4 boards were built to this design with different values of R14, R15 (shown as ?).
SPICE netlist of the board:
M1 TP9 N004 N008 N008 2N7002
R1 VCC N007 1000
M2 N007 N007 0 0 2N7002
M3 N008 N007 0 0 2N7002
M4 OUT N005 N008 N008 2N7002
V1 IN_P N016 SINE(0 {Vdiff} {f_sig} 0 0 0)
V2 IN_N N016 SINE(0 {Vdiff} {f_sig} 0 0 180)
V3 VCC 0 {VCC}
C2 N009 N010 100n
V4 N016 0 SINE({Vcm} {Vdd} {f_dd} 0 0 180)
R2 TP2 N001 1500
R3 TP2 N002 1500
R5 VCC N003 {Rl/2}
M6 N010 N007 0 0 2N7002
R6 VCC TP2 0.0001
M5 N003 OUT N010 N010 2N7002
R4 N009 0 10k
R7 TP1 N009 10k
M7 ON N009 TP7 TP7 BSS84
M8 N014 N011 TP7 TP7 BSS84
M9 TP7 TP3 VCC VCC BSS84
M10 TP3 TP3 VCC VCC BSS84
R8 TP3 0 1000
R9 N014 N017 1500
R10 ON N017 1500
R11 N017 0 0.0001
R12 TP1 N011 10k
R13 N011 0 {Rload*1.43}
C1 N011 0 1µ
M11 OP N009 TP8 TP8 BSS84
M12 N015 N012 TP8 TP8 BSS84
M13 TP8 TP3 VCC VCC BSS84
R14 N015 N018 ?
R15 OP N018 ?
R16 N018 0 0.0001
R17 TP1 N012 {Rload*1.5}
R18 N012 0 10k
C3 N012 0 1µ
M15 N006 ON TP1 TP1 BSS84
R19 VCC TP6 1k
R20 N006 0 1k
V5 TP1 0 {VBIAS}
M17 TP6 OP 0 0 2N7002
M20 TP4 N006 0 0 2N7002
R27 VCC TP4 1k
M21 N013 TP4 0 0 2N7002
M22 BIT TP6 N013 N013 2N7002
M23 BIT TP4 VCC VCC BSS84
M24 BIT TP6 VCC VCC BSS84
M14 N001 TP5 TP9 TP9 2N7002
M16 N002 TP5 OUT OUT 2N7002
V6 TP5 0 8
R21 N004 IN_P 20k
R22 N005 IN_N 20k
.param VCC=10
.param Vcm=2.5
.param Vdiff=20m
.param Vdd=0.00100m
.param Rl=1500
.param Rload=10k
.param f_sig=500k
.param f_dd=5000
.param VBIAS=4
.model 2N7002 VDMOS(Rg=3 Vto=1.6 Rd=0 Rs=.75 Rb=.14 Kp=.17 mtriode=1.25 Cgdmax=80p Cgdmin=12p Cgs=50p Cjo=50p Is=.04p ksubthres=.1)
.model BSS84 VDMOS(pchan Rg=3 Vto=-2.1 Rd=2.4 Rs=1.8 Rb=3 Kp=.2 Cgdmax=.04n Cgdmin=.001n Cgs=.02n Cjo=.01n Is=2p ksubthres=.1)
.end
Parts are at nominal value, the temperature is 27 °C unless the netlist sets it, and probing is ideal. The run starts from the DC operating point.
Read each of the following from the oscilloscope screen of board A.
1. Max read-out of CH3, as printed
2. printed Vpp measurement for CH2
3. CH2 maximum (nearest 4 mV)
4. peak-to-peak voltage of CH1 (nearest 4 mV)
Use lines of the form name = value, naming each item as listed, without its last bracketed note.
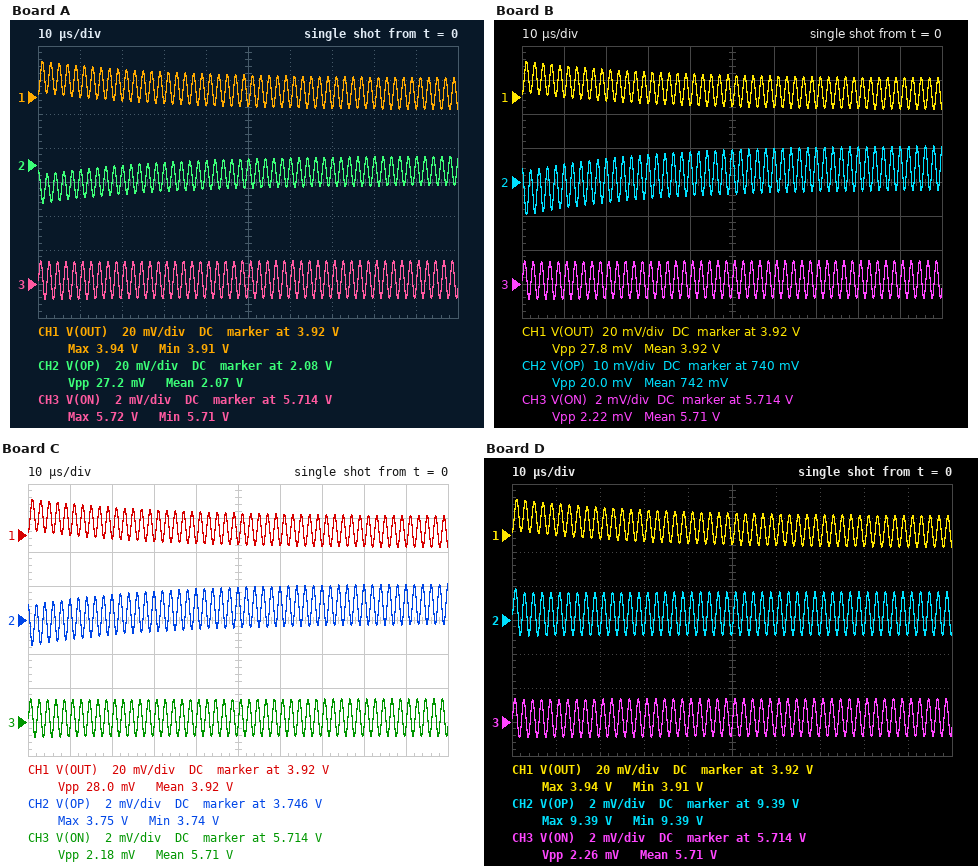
Max read-out of CH3, as printed = 5.72 V
printed Vpp measurement for CH2 = 27.2 mV
CH2 maximum = 2.084 V
peak-to-peak voltage of CH1 = 28 mV
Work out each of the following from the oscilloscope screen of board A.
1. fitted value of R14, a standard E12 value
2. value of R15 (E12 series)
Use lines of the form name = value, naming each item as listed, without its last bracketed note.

fitted value of R14, a standard E12 value = 820 Ω
value of R15 = 820 Ω
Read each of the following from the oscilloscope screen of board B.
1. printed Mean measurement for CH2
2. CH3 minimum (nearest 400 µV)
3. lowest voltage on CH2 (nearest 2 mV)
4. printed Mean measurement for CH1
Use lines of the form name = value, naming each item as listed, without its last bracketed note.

printed Mean measurement for CH2 = 742 mV
CH3 minimum = 5.7132 V
lowest voltage on CH2 = 730 mV
printed Mean measurement for CH1 = 3.92 V
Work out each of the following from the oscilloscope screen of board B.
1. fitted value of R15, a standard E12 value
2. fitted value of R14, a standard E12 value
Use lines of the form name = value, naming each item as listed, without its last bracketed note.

fitted value of R15, a standard E12 value = 470 Ω
fitted value of R14, a standard E12 value = 680 Ω
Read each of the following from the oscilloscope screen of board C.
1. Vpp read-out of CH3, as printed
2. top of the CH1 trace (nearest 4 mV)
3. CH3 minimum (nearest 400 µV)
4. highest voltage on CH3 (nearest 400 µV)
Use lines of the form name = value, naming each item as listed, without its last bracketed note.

Vpp read-out of CH3, as printed = 2.18 mV
top of the CH1 trace = 3.940 V
CH3 minimum = 5.7132 V
highest voltage on CH3 = 5.7152 V
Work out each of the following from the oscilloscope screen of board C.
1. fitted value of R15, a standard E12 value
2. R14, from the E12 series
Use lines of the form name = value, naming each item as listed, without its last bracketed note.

fitted value of R15, a standard E12 value = 560 Ω
R14, from the E12 series = 4.7 kΩ
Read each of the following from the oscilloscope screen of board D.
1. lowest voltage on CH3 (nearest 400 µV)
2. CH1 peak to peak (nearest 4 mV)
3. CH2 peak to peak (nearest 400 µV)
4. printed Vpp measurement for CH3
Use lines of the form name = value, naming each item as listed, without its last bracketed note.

lowest voltage on CH3 = 5.7132 V
CH1 peak to peak = 28 mV
CH2 peak to peak = 2.8 mV
printed Vpp measurement for CH3 = 2.26 mV
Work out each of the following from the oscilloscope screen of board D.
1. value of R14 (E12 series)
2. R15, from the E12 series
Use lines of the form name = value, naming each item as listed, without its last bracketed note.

value of R14 = 1.8 kΩ
R15, from the E12 series = 3.9 kΩ
